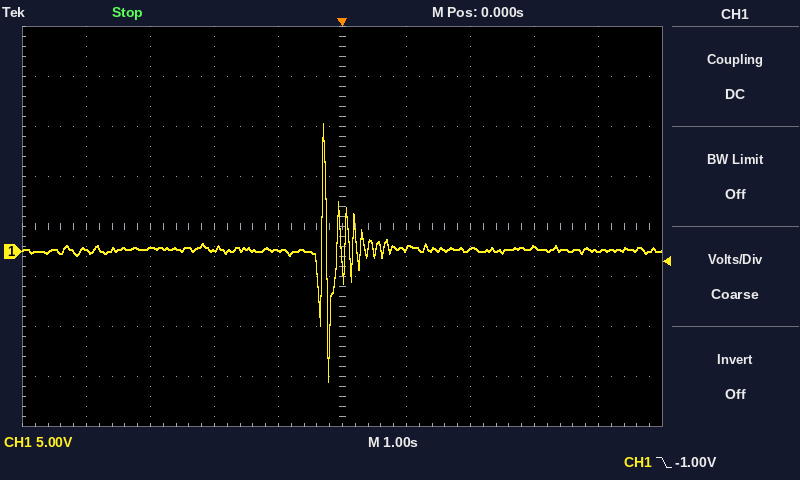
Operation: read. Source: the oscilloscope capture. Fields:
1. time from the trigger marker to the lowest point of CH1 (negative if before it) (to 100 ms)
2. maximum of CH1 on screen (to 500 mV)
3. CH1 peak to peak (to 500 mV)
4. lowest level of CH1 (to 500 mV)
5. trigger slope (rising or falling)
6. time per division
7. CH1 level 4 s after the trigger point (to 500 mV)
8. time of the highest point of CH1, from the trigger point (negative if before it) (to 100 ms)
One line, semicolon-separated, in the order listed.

-200 ms; 13.0 V; 26.0 V; -13.0 V; falling; 1 s; 0.0 V; -300 ms
